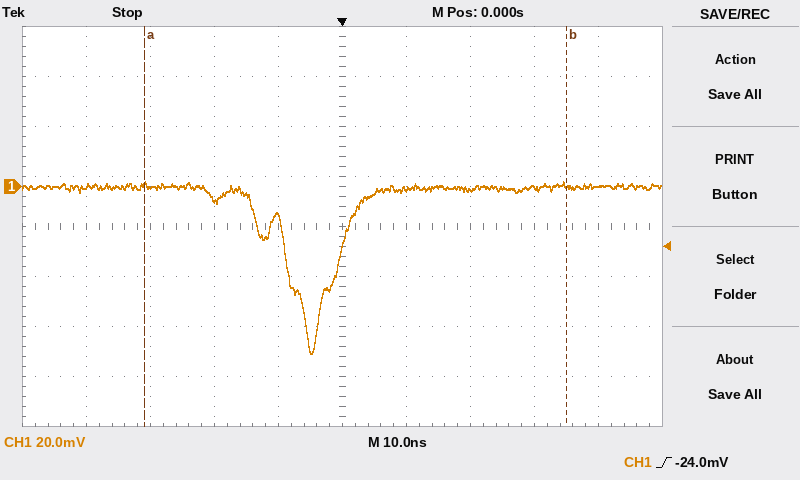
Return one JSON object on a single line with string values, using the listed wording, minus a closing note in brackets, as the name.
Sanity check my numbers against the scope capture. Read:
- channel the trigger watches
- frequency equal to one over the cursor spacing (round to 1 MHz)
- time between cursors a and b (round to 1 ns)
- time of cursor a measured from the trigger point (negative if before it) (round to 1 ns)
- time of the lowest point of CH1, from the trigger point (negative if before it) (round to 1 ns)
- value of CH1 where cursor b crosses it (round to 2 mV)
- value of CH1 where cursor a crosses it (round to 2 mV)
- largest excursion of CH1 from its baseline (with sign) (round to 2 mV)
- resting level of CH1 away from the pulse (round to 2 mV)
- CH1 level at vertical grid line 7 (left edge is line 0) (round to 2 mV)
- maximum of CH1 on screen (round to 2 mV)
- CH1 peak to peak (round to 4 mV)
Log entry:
{"channel the trigger watches": "CH1", "frequency equal to one over the cursor spacing": "15 MHz", "time between cursors a and b": "66 ns", "time of cursor a measured from the trigger point (negative if before it)": "-31 ns", "time of the lowest point of CH1, from the trigger point (negative if before it)": "-5 ns", "value of CH1 where cursor b crosses it": "0 mV", "value of CH1 where cursor a crosses it": "0 mV", "largest excursion of CH1 from its baseline (with sign)": "-66 mV", "resting level of CH1 away from the pulse": "0 mV", "CH1 level at vertical grid line 7 (left edge is line 0)": "-2 mV", "maximum of CH1 on screen": "2 mV", "CH1 peak to peak": "68 mV"}
